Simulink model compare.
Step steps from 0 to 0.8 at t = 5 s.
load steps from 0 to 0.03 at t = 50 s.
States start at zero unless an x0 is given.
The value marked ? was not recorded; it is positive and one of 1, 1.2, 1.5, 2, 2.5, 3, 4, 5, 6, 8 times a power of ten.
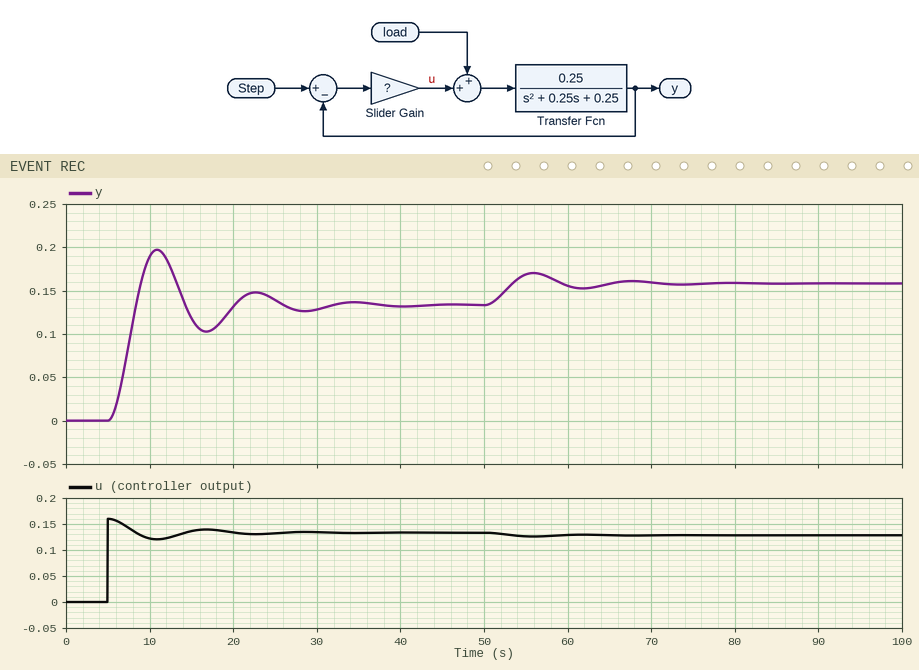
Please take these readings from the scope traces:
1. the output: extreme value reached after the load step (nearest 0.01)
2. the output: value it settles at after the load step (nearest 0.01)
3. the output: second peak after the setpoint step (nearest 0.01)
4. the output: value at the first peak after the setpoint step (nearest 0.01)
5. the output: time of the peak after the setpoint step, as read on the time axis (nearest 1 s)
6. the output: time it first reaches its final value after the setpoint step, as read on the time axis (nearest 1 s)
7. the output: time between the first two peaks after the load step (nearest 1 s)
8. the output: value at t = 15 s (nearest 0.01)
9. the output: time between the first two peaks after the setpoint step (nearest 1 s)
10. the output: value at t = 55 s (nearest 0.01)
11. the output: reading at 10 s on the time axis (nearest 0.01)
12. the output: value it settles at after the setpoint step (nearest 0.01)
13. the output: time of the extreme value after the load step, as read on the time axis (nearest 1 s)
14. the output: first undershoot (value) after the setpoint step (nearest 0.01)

0.17
0.16
0.15
0.20
11 s
8 s
12 s
0.12
12 s
0.17
0.19
0.13
56 s
0.10
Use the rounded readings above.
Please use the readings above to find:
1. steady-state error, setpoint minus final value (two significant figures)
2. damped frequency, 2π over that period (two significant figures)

0.67
0.52 rad/s
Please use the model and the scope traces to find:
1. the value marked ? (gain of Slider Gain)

0.2
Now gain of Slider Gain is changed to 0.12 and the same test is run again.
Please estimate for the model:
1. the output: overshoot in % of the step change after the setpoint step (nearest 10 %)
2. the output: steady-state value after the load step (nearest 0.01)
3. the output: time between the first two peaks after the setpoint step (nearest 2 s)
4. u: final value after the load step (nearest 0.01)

50 %
0.11
12 s
0.08
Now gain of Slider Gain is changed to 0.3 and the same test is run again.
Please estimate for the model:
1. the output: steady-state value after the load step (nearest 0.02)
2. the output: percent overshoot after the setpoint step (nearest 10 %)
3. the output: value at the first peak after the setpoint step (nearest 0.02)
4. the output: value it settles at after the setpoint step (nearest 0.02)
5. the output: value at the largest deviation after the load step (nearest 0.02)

0.20
50 %
0.28
0.18
0.22
